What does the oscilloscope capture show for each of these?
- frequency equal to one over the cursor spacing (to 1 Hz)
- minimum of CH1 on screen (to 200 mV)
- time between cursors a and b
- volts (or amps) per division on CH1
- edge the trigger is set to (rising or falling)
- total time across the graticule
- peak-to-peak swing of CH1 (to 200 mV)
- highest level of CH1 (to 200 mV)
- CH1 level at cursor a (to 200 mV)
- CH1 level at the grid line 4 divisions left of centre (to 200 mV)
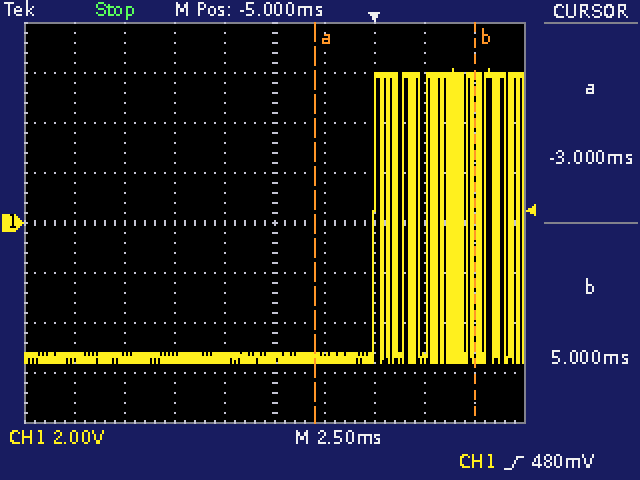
125 Hz
-5.6 V
8.00 ms
2 V
rising
25 ms
11.8 V
6.2 V
-5.4 V
-5.4 V
